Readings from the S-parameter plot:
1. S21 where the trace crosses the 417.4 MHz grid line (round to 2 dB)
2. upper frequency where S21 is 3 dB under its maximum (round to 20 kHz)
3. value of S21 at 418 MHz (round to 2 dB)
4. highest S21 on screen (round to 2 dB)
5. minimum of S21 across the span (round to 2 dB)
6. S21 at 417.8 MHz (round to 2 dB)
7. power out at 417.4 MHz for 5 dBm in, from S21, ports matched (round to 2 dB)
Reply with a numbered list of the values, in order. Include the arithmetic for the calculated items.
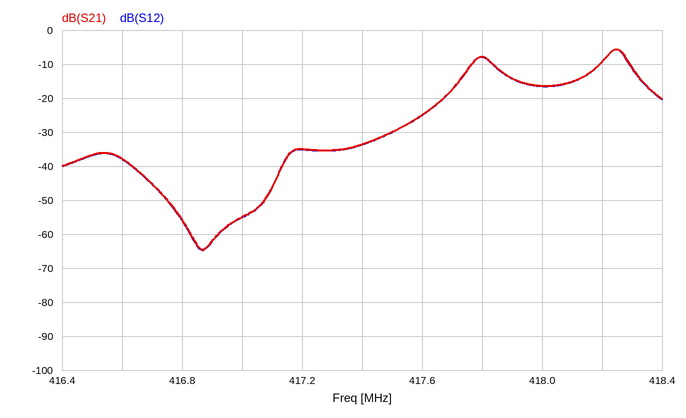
1. -34 dB
2. 418.28 MHz
3. -16 dB
4. -6 dB
5. -64 dB
6. -8 dB
7. 5 dBm + (-34 dB) = -28 dBm
